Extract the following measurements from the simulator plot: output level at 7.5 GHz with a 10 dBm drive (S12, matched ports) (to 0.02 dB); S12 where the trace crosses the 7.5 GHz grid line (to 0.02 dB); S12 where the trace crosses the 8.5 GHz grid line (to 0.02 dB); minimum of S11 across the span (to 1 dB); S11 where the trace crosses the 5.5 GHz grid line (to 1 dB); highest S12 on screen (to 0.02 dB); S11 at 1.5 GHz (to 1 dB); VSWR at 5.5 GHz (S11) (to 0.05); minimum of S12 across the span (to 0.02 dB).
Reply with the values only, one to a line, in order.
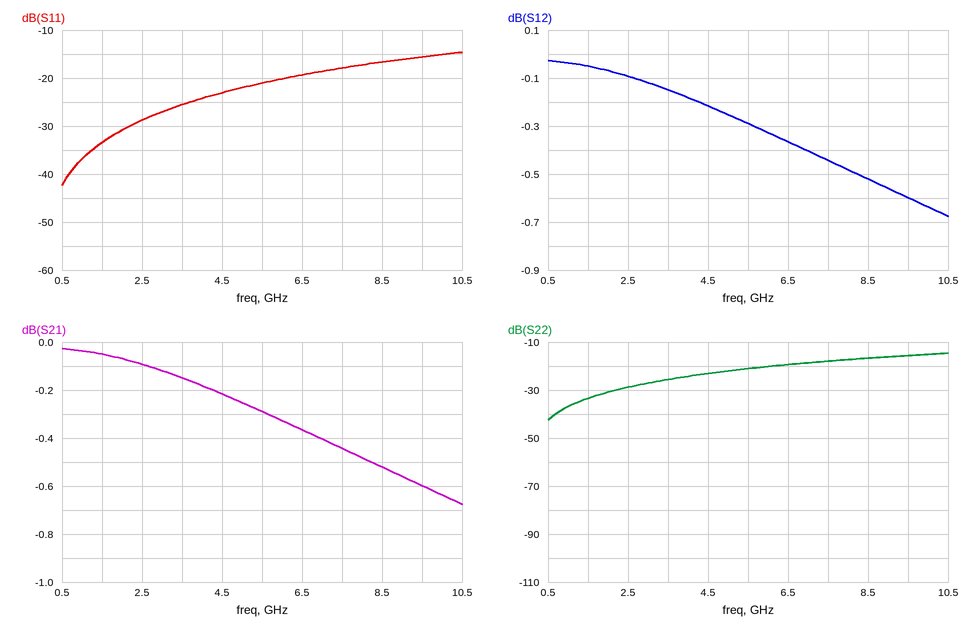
9.56 dBm
-0.44 dB
-0.52 dB
-42 dB
-21 dB
-0.02 dB
-33 dB
1.20
-0.68 dB
